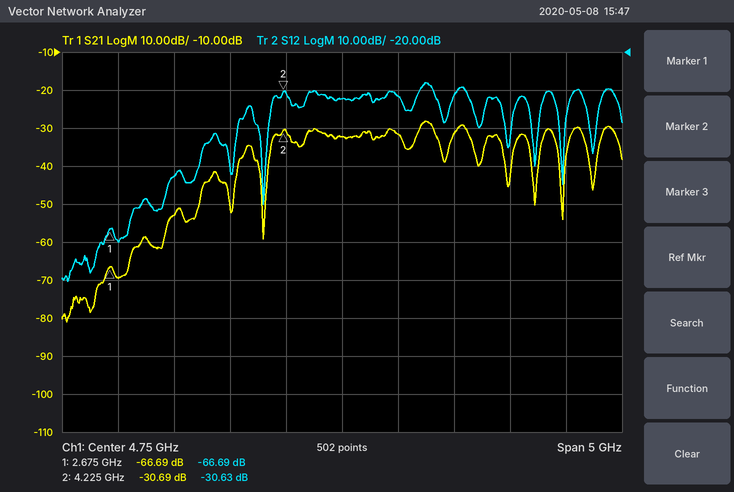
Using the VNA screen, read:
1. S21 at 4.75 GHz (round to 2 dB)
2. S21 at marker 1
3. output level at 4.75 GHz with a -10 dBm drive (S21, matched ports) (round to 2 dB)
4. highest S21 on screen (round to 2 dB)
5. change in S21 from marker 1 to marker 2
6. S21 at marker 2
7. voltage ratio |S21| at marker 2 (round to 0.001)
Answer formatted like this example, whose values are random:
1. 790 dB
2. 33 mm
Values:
1. -32 dB
2. -66.69 dB
3. -42 dBm
4. -28 dB
5. 36.00 dB
6. -30.69 dB
7. 0.029
